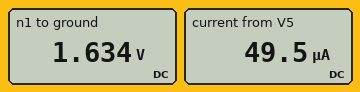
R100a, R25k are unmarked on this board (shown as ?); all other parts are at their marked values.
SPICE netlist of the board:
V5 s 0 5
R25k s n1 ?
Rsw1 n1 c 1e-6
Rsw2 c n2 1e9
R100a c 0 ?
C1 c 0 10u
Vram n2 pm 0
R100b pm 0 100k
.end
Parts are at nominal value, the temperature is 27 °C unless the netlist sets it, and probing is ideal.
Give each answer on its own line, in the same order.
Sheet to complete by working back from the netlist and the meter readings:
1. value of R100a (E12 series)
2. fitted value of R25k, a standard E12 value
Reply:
33 kΩ
68 kΩ
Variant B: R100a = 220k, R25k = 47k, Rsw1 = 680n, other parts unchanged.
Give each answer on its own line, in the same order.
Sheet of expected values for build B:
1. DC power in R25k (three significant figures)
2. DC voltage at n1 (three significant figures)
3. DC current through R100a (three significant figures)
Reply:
16.5 µW
4.12 V
18.7 µA
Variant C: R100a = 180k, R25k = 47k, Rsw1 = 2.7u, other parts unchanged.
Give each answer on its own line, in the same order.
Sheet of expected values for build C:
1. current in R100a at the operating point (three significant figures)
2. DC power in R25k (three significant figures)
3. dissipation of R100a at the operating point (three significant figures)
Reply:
22.0 µA
22.8 µW
87.3 µW
